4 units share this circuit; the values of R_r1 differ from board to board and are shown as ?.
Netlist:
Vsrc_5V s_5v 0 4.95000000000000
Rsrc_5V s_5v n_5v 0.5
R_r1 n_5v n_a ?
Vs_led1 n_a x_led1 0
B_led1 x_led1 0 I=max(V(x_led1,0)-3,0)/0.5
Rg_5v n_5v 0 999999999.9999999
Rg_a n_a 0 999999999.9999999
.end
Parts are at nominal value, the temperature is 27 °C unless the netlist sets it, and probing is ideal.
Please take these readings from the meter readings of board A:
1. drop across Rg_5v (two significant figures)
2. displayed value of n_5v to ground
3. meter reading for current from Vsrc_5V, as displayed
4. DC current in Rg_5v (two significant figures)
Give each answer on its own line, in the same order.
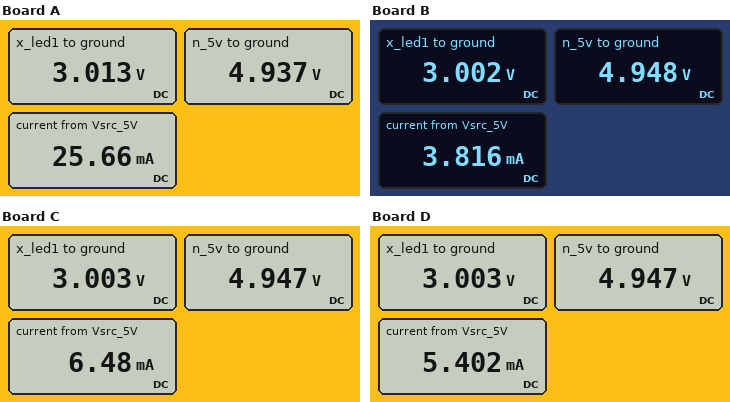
4.9 V
4.937 V
25.66 mA
4.9 nA
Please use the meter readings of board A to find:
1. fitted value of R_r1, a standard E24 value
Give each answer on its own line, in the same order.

75 Ω
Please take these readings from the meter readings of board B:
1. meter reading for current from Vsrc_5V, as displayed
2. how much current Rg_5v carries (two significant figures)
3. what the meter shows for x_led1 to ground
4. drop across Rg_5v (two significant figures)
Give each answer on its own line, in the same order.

3.816 mA
4.9 nA
3.002 V
4.9 V
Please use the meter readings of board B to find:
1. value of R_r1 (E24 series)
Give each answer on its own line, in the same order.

510 Ω
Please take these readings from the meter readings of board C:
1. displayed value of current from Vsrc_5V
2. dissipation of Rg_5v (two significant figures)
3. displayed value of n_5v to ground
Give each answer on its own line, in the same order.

6.48 mA
24 nW
4.947 V
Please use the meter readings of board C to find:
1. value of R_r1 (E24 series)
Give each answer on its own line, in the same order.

300 Ω
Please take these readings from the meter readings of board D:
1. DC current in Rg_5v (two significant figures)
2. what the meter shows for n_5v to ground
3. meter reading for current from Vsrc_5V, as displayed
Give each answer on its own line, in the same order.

4.9 nA
4.947 V
5.402 mA
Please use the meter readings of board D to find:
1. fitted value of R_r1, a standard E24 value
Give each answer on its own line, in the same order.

360 Ω
